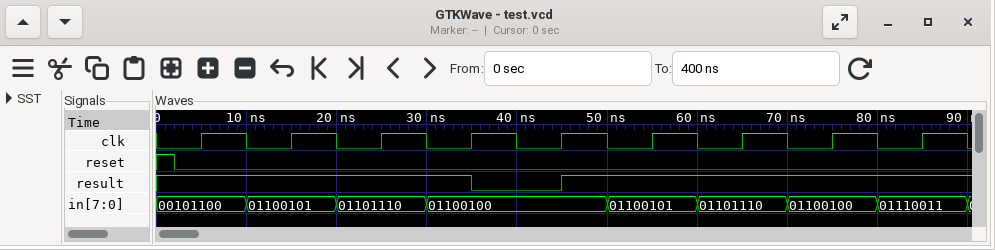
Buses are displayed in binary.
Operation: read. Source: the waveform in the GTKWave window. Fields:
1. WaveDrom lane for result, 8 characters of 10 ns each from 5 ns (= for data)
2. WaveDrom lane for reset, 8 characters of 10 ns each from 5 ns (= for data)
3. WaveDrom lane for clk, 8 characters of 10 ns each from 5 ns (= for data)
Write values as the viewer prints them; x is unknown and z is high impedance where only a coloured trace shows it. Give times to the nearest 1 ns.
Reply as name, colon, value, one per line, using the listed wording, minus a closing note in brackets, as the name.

WaveDrom lane for result, 8 characters of 10 ns each from 5 ns: {name: 'result', wave: '1..01...'}
WaveDrom lane for reset, 8 characters of 10 ns each from 5 ns: {name: 'reset', wave: '0.......'}
WaveDrom lane for clk, 8 characters of 10 ns each from 5 ns: {name: 'clk', wave: 'p.......'}
